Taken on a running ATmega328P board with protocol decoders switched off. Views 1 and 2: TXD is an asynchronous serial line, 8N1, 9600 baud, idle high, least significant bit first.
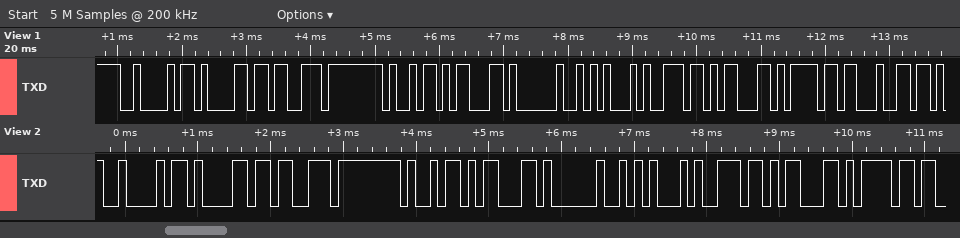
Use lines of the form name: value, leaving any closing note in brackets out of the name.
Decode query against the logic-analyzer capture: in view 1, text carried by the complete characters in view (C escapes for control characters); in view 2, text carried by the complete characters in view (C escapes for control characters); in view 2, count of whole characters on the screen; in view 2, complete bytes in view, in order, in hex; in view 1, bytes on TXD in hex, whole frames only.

in view 1, text carried by the complete characters in view: "Basic Encod"
in view 2, text carried by the complete characters in view: "Basic Enco"
in view 2, count of whole characters on the screen: 10
in view 2, complete bytes in view, in order, in hex: 42 61 73 69 63 20 45 6E 63 6F
in view 1, bytes on TXD in hex, whole frames only: 42 61 73 69 63 20 45 6E 63 6F 64
